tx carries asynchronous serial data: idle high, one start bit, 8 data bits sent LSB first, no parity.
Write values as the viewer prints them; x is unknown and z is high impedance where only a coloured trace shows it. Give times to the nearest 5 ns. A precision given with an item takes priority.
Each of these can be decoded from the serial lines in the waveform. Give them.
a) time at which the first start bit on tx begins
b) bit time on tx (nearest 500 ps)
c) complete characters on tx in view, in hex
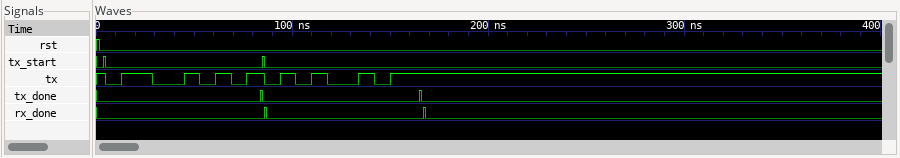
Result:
5 ns
8000 ps
53, A5
